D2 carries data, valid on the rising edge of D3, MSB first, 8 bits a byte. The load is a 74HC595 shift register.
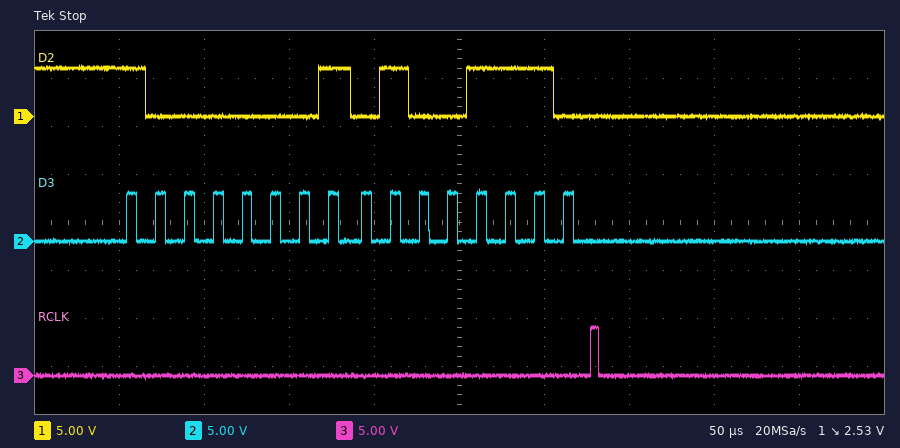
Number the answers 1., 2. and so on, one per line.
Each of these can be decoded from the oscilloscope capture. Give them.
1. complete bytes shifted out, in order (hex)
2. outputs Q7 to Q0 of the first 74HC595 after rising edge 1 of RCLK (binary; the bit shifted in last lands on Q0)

1. 81 4E
2. 01001110
